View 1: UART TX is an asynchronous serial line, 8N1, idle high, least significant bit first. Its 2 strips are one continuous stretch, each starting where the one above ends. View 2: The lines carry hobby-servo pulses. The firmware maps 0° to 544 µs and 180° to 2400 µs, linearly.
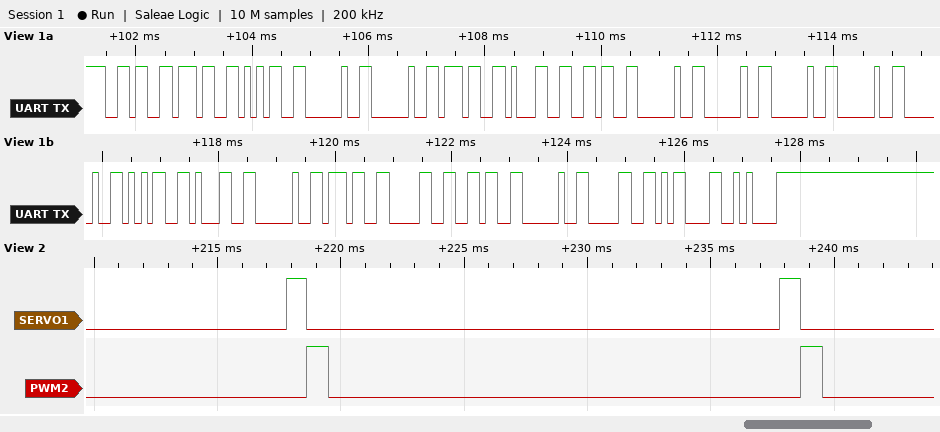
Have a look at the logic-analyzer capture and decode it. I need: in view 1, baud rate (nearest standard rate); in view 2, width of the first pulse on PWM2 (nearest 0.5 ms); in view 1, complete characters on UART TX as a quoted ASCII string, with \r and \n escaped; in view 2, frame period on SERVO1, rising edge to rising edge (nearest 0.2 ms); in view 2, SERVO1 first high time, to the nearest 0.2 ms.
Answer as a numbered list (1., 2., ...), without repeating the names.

1. 9600 baud
2. 1.0 ms
3. "675  716     51 706 0\r\n"
4. 20.0 ms
5. 0.8 ms
